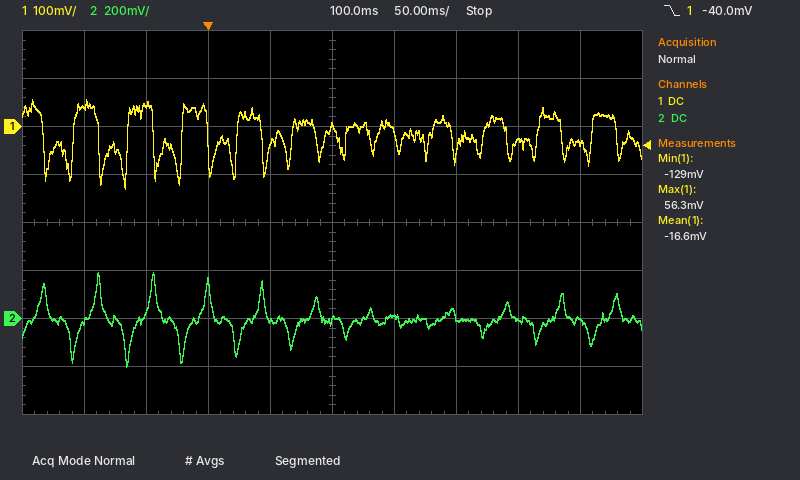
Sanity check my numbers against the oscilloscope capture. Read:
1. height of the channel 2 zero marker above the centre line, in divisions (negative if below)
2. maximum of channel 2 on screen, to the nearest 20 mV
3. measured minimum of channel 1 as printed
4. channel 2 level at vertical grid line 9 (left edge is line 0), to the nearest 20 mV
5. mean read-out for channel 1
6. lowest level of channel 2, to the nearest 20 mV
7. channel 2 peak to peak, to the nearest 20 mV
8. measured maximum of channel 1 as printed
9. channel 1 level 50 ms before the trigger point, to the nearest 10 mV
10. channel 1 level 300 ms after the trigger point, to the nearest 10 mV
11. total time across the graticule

-2.0 div
200 mV
-129 mV
0 mV
-16.6 mV
-200 mV
400 mV
56.3 mV
50 mV
-30 mV
500 ms
